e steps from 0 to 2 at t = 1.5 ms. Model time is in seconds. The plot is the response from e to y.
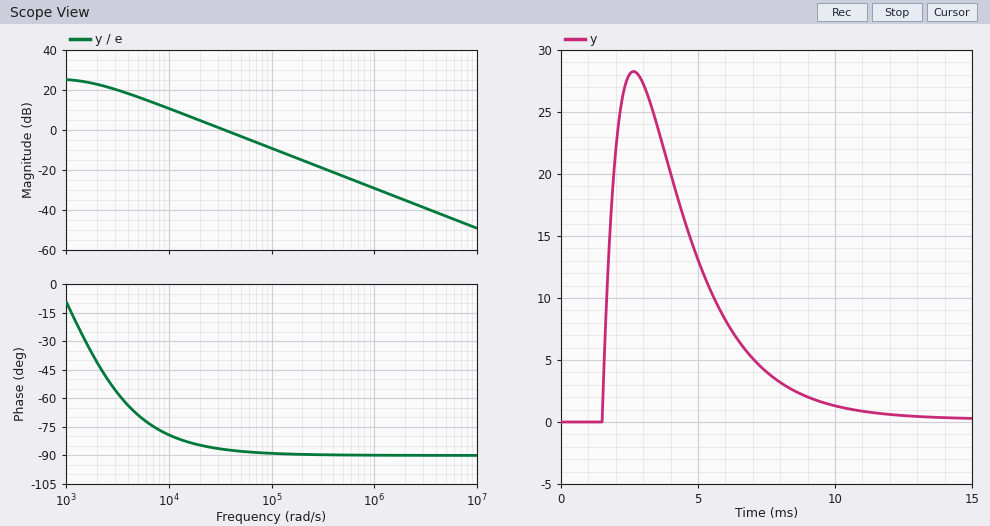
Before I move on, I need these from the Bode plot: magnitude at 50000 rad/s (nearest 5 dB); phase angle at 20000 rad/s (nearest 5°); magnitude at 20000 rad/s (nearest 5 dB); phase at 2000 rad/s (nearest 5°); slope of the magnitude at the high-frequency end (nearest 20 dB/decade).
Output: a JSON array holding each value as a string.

["-5 dB", "-85°", "5 dB", "-40°", "-20 dB/decade"]
